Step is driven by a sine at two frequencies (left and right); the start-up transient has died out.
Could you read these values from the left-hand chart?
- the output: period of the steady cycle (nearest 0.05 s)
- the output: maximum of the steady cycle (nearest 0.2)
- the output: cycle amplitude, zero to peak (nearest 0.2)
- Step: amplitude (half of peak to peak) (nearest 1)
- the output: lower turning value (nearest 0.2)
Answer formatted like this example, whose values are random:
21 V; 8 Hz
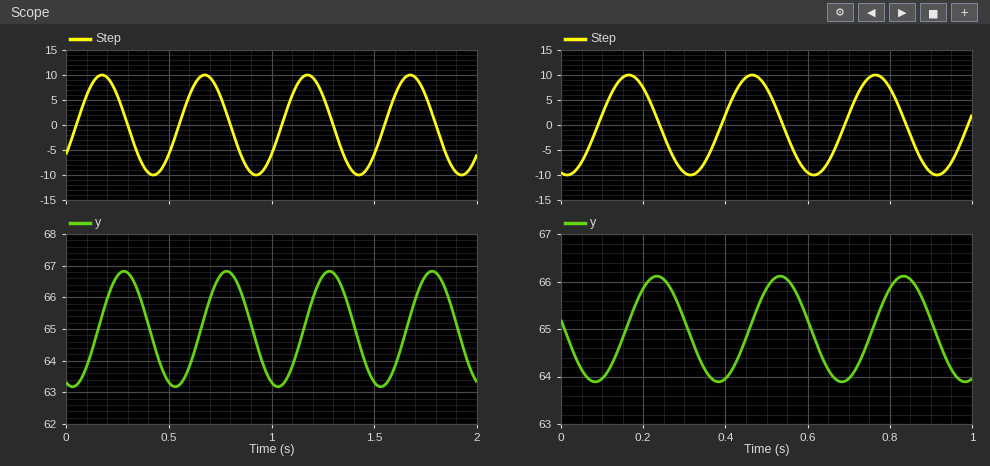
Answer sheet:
0.50 s; 66.8; 1.8; 10; 63.2
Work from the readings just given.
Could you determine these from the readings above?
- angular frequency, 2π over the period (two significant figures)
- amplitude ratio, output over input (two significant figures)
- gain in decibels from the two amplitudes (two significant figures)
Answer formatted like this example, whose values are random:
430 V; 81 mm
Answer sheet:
13 rad/s; 0.18; -15 dB
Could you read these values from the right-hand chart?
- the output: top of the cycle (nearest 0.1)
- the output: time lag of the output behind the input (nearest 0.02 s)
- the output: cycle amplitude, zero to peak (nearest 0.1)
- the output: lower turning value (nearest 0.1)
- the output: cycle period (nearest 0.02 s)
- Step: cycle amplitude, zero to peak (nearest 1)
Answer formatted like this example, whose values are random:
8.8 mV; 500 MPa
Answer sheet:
66.1; 0.06 s; 1.1; 63.9; 0.30 s; 10
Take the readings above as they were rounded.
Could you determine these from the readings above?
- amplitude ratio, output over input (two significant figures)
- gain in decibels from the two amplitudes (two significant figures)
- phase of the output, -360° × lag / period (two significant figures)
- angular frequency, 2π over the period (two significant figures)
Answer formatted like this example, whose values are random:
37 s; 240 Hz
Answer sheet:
0.11; -19 dB; -72°; 21 rad/s
